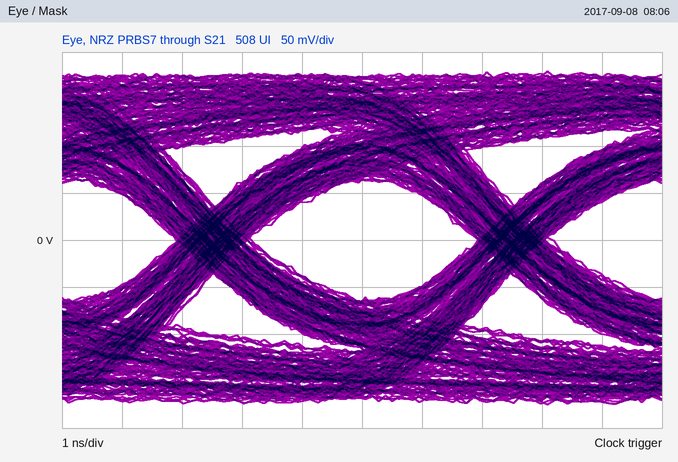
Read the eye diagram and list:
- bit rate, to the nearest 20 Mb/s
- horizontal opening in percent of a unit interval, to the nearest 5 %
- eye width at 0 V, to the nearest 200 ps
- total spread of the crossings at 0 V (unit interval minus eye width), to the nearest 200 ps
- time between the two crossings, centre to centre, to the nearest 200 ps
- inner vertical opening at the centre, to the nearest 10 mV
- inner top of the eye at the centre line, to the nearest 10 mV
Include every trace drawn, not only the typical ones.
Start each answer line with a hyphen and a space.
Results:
- 200 Mb/s
- 75 %
- 3.8 ns
- 1.2 ns
- 5.0 ns
- 130 mV
- 60 mV
